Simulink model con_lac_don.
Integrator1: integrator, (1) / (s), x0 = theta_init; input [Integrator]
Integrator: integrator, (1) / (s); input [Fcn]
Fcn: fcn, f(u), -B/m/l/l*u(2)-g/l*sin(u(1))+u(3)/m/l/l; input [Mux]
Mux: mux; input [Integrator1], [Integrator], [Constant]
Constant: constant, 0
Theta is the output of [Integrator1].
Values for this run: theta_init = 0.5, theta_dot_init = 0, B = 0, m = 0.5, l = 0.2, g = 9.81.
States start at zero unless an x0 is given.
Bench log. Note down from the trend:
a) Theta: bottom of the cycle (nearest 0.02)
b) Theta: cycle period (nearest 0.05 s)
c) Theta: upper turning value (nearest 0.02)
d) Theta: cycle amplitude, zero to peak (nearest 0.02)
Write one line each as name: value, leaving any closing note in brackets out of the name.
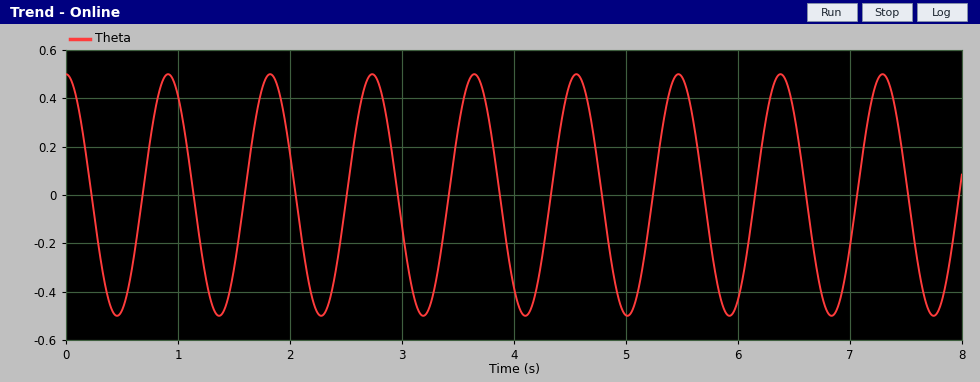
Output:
Theta: bottom of the cycle: -0.50
Theta: cycle period: 0.90 s
Theta: upper turning value: 0.50
Theta: cycle amplitude, zero to peak: 0.50
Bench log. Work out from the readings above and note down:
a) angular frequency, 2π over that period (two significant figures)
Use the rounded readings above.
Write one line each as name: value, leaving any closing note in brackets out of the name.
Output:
angular frequency, 2π over that period: 7.0 rad/s
